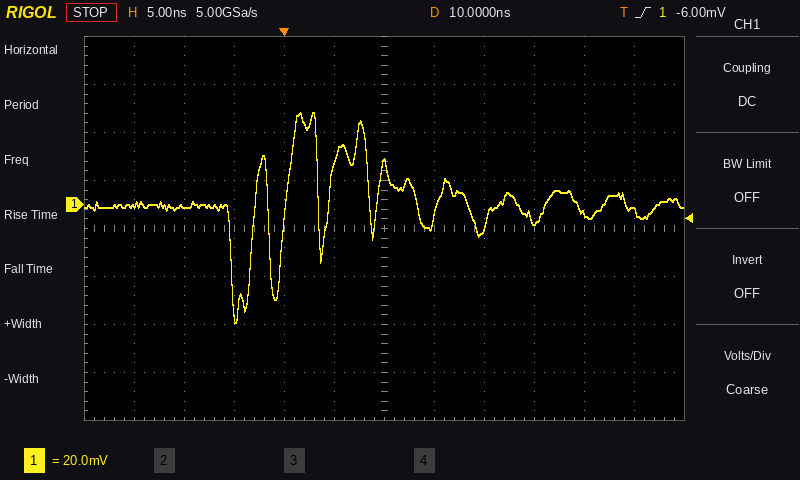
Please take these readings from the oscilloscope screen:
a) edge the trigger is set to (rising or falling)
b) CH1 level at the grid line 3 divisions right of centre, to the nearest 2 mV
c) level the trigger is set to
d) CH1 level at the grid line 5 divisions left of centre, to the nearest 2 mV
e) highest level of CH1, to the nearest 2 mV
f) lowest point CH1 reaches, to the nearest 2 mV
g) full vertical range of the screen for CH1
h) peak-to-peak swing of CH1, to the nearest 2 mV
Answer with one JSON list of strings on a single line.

["rising", "-8 mV", "-6.00 mV", "0 mV", "38 mV", "-50 mV", "160 mV", "88 mV"]
